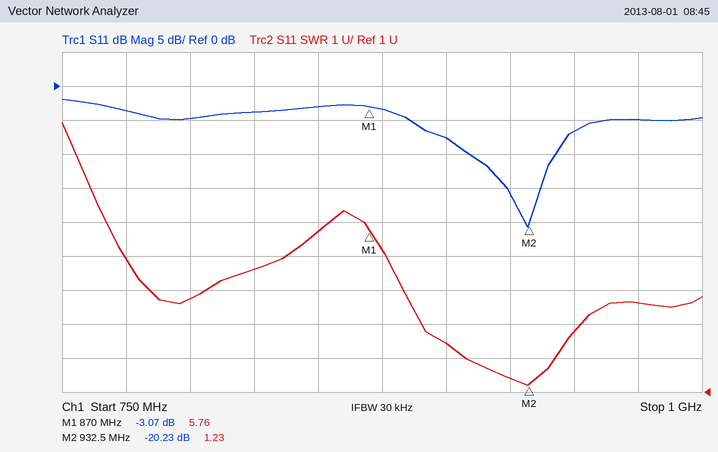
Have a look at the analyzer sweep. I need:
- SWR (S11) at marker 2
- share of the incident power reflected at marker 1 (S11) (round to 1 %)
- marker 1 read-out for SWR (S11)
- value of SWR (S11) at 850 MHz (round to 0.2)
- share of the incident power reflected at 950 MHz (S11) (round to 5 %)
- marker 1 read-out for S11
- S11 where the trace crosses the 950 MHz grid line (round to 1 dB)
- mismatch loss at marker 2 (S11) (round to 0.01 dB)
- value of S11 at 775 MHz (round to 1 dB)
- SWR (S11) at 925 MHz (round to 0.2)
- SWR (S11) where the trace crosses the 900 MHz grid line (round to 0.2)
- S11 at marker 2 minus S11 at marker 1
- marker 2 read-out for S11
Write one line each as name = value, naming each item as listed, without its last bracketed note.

SWR (S11) at marker 2 = 1.23
share of the incident power reflected at marker 1 (S11) = 49 %
marker 1 read-out for SWR = 5.76
value of SWR (S11) at 850 MHz = 5.8
share of the incident power reflected at 950 MHz (S11) = 20 %
marker 1 read-out for S11 = -3.07 dB
S11 where the trace crosses the 950 MHz grid line = -7 dB
mismatch loss at marker 2 (S11) = 0.04 dB
value of S11 at 775 MHz = -4 dB
SWR (S11) at 925 MHz = 1.4
SWR (S11) where the trace crosses the 900 MHz grid line = 2.4
S11 at marker 2 minus S11 at marker 1 = -17.16 dB
marker 2 read-out for S11 = -20.23 dB
